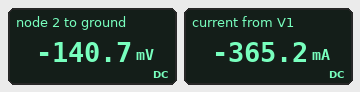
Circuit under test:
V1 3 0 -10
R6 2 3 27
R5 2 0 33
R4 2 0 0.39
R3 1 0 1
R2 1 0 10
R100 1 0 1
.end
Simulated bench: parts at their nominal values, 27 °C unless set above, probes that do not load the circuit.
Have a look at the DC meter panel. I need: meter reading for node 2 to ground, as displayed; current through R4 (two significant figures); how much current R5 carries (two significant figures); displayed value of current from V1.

-140.7 mV
360 mA
4.3 mA
-365.2 mA
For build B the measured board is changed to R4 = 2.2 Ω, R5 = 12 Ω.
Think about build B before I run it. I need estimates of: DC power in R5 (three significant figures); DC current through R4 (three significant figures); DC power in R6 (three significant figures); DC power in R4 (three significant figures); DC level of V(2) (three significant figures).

34.6 mW
293 mA
3.24 W
189 mW
-644 mV
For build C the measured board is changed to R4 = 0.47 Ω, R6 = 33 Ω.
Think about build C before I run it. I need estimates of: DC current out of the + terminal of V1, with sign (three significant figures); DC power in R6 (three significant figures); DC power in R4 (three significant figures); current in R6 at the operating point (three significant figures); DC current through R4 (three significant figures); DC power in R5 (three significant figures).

-299 mA
2.95 W
40.8 mW
299 mA
295 mA
581 µW
